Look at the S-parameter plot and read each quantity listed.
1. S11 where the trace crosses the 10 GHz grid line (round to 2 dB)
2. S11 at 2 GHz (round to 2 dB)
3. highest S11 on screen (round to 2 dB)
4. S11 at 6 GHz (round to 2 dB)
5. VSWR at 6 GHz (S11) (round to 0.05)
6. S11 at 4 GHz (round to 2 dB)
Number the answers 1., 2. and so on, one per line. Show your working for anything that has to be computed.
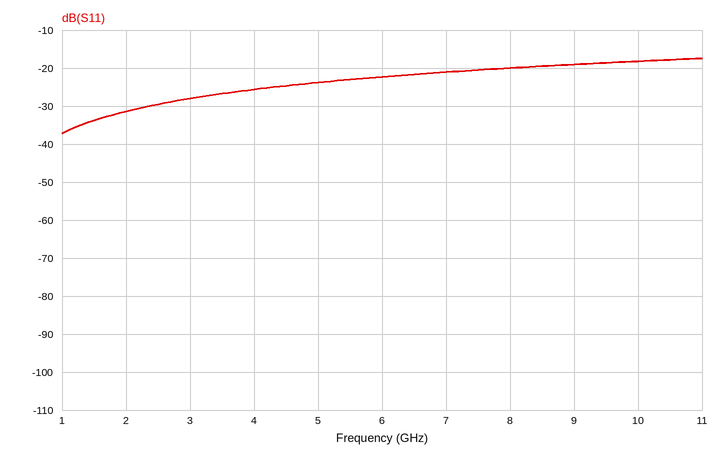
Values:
1. -18 dB
2. -32 dB
3. -18 dB
4. -22 dB
5. |Γ| = 10^(-22/20) = 0.0794; VSWR = (1 + 0.0794)/(1 − 0.0794) ≈ 1.17, so 1.15 to the nearest 0.05
6. -26 dB
